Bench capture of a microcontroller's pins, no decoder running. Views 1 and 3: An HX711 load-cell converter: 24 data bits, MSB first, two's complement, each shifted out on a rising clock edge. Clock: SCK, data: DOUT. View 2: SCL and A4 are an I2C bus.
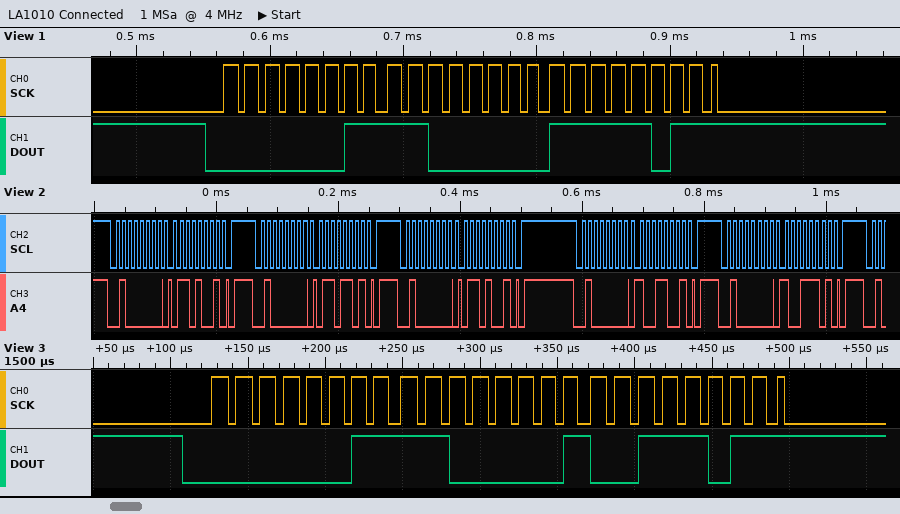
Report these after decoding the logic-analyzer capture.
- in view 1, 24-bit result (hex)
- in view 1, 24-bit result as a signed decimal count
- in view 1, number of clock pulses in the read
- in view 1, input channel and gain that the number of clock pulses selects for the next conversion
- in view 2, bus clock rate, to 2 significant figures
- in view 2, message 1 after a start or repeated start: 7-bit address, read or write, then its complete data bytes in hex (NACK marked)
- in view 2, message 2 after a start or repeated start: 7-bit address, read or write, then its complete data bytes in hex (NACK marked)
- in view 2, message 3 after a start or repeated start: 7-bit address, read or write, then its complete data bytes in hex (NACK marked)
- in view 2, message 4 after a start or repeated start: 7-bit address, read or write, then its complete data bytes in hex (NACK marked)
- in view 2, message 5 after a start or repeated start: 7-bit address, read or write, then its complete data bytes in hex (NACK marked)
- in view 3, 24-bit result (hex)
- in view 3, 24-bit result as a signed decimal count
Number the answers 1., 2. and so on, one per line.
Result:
1. 0x03C0FB
2. 246011
3. 25
4. channel A, gain 128
5. 100 kHz
6. 0x20 write: 69
7. 0x20 write: 6D
8. 0x20 write: 69
9. 0x20 write: 99
10. 0x20 write: 9D
11. 0x03C13B
12. 246075
